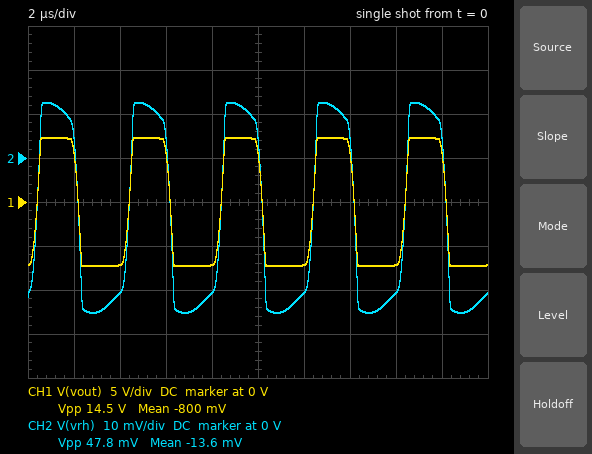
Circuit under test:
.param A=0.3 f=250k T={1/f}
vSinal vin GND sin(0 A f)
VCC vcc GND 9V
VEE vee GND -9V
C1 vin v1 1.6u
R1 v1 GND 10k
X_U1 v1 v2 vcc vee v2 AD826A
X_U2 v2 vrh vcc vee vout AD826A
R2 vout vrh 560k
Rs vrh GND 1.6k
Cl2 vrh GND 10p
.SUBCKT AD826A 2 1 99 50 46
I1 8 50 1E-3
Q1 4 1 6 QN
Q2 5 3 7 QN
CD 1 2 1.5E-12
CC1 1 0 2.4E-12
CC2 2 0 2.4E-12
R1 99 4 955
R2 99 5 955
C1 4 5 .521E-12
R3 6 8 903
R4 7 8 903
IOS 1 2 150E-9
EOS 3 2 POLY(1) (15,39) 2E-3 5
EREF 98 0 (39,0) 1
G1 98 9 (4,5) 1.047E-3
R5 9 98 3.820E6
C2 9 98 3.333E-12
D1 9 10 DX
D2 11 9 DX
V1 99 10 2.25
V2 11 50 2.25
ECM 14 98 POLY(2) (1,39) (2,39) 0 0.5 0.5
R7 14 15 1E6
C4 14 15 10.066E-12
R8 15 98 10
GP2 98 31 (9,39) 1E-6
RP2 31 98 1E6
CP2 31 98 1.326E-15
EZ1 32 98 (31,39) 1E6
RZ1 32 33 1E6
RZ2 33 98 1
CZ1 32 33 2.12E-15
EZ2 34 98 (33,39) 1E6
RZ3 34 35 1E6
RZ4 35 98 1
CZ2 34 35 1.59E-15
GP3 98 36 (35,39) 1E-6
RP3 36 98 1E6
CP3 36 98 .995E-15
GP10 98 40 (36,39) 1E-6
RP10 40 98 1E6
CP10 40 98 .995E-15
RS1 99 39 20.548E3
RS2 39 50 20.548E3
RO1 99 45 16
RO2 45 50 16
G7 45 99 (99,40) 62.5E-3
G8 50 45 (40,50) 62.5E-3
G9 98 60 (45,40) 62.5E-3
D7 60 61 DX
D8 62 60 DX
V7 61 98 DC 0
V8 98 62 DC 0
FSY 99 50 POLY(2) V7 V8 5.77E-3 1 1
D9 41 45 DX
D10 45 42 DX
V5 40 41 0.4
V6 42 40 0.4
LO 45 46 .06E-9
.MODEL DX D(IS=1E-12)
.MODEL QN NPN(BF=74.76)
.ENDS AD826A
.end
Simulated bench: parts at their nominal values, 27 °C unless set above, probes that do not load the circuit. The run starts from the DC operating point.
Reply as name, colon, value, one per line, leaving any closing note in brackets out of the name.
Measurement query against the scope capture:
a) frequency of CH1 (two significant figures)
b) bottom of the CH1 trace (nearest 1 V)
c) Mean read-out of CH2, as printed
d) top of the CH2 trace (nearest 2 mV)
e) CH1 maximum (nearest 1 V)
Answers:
frequency of CH1: 250 kHz
bottom of the CH1 trace: -7 V
Mean read-out of CH2, as printed: -13.6 mV
top of the CH2 trace: 12 mV
CH1 maximum: 7 V
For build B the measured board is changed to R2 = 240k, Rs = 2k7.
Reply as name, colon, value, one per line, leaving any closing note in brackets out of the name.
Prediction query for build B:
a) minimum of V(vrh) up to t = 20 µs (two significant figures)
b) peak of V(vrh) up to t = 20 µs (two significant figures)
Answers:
minimum of V(vrh) up to t = 20 µs: -100 mV
peak of V(vrh) up to t = 20 µs: 66 mV
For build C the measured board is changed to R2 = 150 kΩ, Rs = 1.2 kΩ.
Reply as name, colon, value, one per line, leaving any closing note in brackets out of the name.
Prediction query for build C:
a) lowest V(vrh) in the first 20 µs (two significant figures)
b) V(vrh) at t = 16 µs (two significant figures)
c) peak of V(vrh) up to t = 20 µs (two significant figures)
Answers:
lowest V(vrh) in the first 20 µs: -68 mV
V(vrh) at t = 16 µs: -64 mV
peak of V(vrh) up to t = 20 µs: 51 mV
